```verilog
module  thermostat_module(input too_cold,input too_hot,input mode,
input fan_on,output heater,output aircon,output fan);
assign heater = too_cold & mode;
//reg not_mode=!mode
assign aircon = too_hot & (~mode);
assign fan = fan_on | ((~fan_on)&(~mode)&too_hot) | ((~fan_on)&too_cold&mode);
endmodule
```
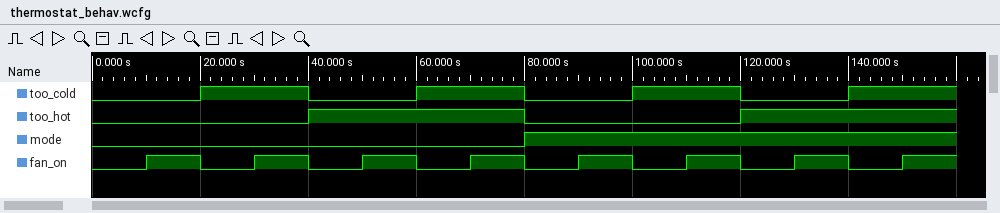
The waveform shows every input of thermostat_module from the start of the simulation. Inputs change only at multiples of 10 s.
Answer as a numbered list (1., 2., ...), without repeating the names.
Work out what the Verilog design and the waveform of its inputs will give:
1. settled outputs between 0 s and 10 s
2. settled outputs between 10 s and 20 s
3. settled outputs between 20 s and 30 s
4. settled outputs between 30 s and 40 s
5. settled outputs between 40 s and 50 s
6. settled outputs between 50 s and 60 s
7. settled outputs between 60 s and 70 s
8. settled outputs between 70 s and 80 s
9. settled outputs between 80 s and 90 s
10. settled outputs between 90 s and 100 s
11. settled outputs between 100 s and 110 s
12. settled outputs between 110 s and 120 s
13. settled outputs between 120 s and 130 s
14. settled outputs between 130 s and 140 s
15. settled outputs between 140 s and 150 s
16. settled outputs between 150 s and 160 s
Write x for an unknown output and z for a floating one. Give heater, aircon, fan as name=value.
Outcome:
1. heater=0, aircon=0, fan=0
2. heater=0, aircon=0, fan=1
3. heater=0, aircon=0, fan=0
4. heater=0, aircon=0, fan=1
5. heater=0, aircon=1, fan=1
6. heater=0, aircon=1, fan=1
7. heater=0, aircon=1, fan=1
8. heater=0, aircon=1, fan=1
9. heater=0, aircon=0, fan=0
10. heater=0, aircon=0, fan=1
11. heater=1, aircon=0, fan=1
12. heater=1, aircon=0, fan=1
13. heater=0, aircon=0, fan=0
14. heater=0, aircon=0, fan=1
15. heater=1, aircon=0, fan=1
16. heater=1, aircon=0, fan=1
